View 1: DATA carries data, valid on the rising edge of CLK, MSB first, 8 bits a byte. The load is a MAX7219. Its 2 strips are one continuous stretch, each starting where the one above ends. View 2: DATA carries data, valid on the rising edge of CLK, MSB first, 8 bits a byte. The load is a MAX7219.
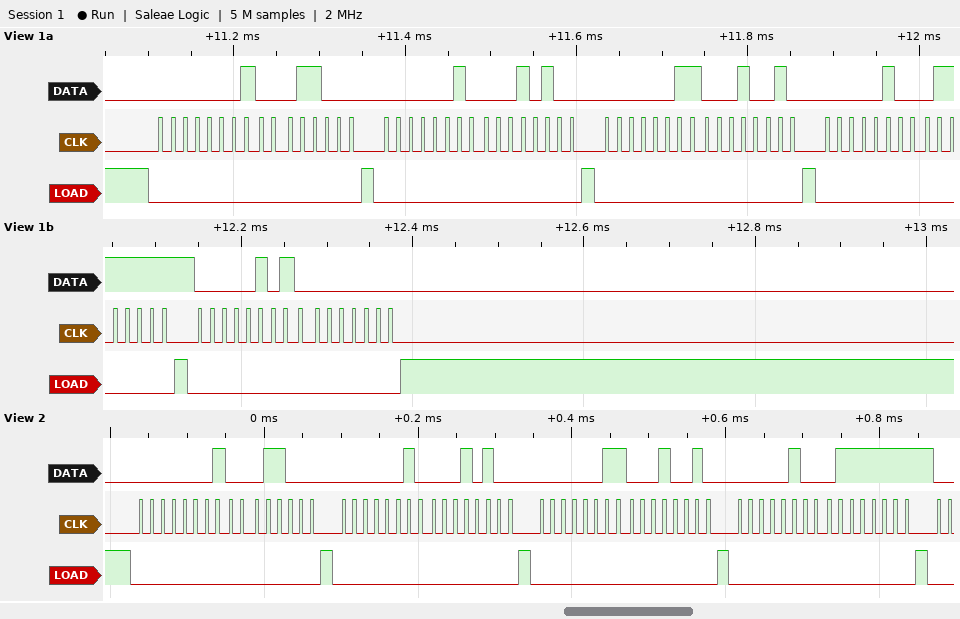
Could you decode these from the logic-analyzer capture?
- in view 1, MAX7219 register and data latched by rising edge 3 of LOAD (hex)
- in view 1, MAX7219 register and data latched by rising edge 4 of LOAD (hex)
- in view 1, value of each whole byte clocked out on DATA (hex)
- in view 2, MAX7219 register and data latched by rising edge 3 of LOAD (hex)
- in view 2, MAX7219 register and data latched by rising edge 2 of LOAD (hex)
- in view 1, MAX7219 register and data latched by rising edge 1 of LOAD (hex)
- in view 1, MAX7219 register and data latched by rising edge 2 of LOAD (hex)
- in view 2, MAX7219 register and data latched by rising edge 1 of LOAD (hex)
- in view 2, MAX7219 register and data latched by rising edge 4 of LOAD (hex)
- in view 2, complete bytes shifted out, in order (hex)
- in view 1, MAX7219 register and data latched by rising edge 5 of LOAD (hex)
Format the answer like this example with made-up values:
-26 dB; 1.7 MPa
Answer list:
register 0x3, data 0x12; register 0x4, data 0x7F; 0x01 0x18 0x02 0x14 0x03 0x12 0x04 0x7F 0x05 0x00; register 0x3, data 0x12; register 0x2, data 0x14; register 0x1, data 0x18; register 0x2, data 0x14; register 0x1, data 0x18; register 0x4, data 0x7F; 01 18 02 14 03 12 04 7F; register 0x5, data 0x00
